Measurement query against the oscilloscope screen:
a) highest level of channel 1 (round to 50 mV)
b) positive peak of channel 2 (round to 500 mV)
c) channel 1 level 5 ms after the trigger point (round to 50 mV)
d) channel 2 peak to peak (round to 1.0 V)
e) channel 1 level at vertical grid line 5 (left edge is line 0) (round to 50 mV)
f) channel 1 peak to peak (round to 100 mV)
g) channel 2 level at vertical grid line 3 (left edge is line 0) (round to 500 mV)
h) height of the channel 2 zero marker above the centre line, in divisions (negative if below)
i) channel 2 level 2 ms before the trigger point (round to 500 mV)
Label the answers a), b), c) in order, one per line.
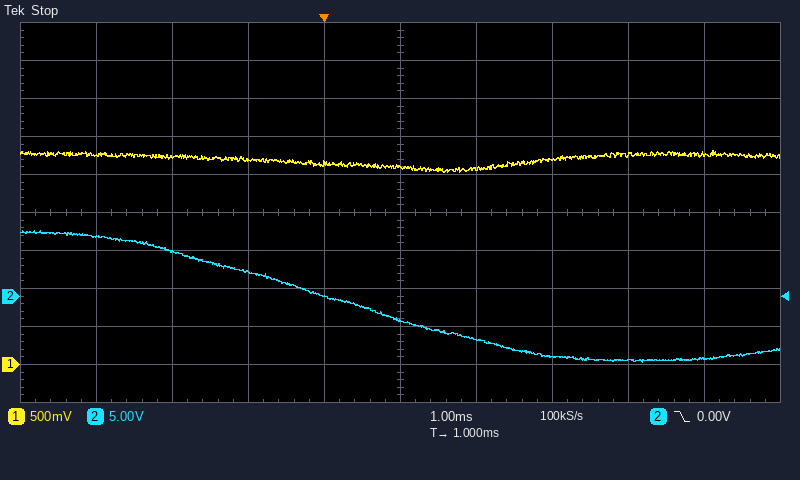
a) 2.80 V
b) 8.5 V
c) 2.75 V
d) 17.0 V
e) 2.60 V
f) 300 mV
g) 3.0 V
h) -2.2 div
i) 6.0 V
